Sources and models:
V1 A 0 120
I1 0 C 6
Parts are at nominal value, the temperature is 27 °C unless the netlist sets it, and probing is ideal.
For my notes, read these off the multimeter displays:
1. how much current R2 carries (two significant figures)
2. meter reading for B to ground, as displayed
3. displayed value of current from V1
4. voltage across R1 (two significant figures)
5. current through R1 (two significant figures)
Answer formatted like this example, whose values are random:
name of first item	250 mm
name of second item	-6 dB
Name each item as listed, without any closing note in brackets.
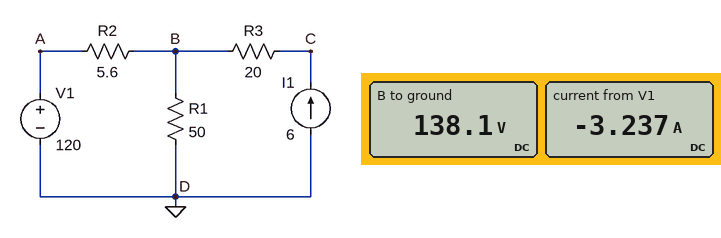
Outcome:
how much current R2 carries	3.2 A
meter reading for B to ground, as displayed	138.1 V
displayed value of current from V1	-3.237 A
voltage across R1	140 V
current through R1	2.8 A
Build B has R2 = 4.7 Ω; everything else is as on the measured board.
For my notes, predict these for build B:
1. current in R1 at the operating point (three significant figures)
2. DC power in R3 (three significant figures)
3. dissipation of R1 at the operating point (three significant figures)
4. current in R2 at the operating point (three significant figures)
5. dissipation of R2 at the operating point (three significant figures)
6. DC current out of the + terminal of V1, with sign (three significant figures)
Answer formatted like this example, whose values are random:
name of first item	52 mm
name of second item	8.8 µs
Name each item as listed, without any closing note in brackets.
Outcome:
current in R1 at the operating point	2.71 A
DC power in R3	720 W
dissipation of R1 at the operating point	367 W
current in R2 at the operating point	3.29 A
dissipation of R2 at the operating point	50.9 W
DC current out of the + terminal of V1, with sign	-3.29 A
